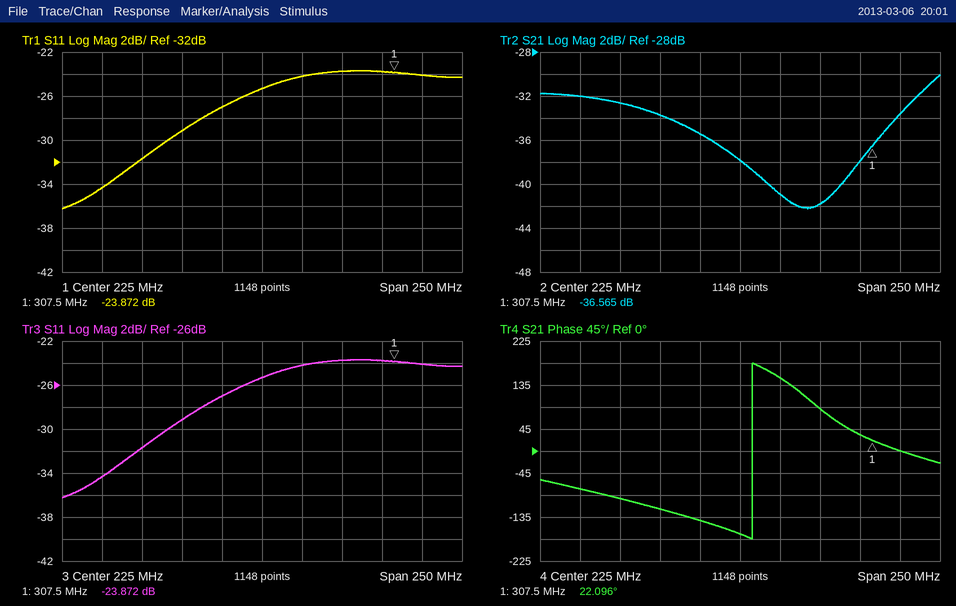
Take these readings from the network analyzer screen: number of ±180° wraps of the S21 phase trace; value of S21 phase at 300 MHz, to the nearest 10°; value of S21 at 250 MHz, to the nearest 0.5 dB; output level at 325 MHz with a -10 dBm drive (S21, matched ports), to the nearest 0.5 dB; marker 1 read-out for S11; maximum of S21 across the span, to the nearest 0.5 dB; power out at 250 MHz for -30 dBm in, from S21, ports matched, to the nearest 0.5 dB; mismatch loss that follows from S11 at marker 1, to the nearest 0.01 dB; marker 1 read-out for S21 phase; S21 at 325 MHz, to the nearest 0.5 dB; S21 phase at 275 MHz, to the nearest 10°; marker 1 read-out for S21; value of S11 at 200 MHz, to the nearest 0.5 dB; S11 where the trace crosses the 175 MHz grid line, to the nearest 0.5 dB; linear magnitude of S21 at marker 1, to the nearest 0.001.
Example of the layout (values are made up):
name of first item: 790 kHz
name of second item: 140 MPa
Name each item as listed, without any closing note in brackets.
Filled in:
number of ±180° wraps of the S21 phase trace: 1
value of S21 phase at 300 MHz, to the nearest 10°: 30°
value of S21 at 250 MHz, to the nearest 0.5 dB: -41.0 dB
output level at 325 MHz with a -10 dBm drive (S21, matched ports), to the nearest 0.5 dB: -43.5 dBm
marker 1 read-out for S11: -23.872 dB
maximum of S21 across the span, to the nearest 0.5 dB: -30.0 dB
power out at 250 MHz for -30 dBm in, from S21, ports matched, to the nearest 0.5 dB: -71.0 dBm
mismatch loss that follows from S11 at marker 1, to the nearest 0.01 dB: 0.02 dB
marker 1 read-out for S21 phase: 22.096°
S21 at 325 MHz, to the nearest 0.5 dB: -33.5 dB
S21 phase at 275 MHz, to the nearest 10°: 90°
marker 1 read-out for S21: -36.565 dB
value of S11 at 200 MHz, to the nearest 0.5 dB: -27.0 dB
S11 where the trace crosses the 175 MHz grid line, to the nearest 0.5 dB: -29.0 dB
linear magnitude of S21 at marker 1, to the nearest 0.001: 0.015
